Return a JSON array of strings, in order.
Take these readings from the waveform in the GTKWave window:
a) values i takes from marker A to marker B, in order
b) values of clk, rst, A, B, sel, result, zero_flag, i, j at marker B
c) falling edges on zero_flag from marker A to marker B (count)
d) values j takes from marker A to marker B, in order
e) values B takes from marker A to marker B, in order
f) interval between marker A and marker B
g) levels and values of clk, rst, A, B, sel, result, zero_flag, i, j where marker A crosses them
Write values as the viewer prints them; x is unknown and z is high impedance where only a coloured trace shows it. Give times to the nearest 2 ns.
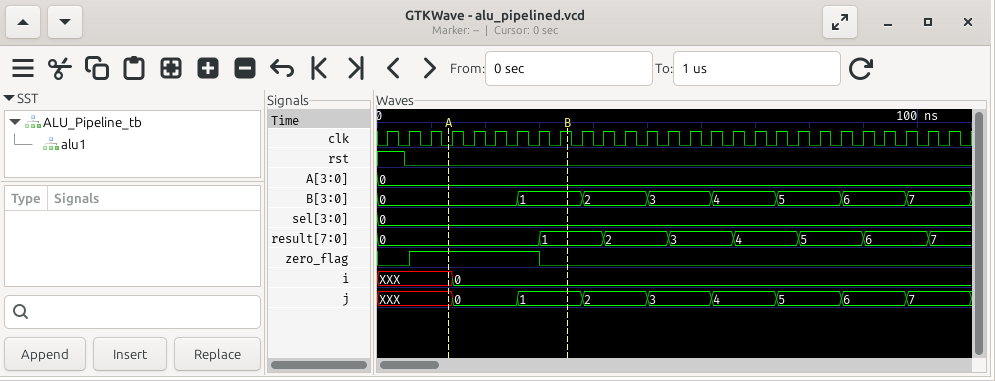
["XXX, 0", "clk=1, rst=0, A=0, B=1, sel=0, result=1, zero_flag=0, i=0, j=1", "1", "XXX, 0, 1", "0, 1", "22 ns", "clk=0, rst=0, A=0, B=0, sel=0, result=0, zero_flag=1, i=XXX, j=XXX"]
